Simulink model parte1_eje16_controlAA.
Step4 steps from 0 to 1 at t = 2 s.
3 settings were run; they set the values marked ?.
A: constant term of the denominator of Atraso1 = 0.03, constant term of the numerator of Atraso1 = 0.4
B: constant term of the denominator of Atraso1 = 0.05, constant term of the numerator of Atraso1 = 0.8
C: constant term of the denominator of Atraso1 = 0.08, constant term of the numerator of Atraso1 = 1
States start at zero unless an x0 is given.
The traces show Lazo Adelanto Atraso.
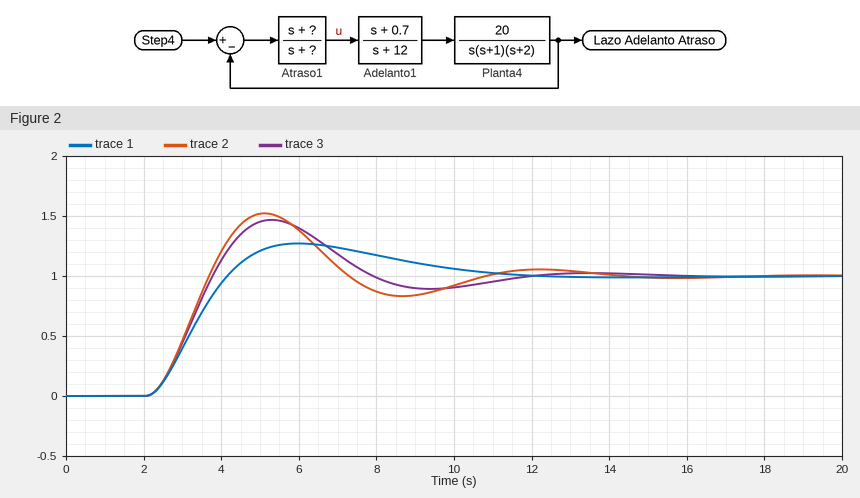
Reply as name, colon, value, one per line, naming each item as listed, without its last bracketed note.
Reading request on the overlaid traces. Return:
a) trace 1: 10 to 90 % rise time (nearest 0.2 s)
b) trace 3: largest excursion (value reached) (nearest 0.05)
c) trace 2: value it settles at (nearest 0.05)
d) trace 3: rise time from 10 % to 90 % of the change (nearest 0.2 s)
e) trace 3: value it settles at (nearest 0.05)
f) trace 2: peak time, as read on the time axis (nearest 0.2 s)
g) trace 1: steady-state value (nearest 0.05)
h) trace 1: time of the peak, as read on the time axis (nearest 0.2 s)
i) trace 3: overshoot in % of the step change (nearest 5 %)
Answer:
trace 1: 10 to 90 % rise time: 1.4 s
trace 3: largest excursion (value reached): 1.45
trace 2: value it settles at: 1.00
trace 3: rise time from 10 % to 90 % of the change: 1.2 s
trace 3: value it settles at: 1.00
trace 2: peak time, as read on the time axis: 5.2 s
trace 1: steady-state value: 1.00
trace 1: time of the peak, as read on the time axis: 6.0 s
trace 3: overshoot in % of the step change: 45 %
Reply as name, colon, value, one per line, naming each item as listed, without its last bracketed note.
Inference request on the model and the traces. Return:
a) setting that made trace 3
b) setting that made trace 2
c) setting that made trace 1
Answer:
setting that made trace 3: B
setting that made trace 2: C
setting that made trace 1: A
